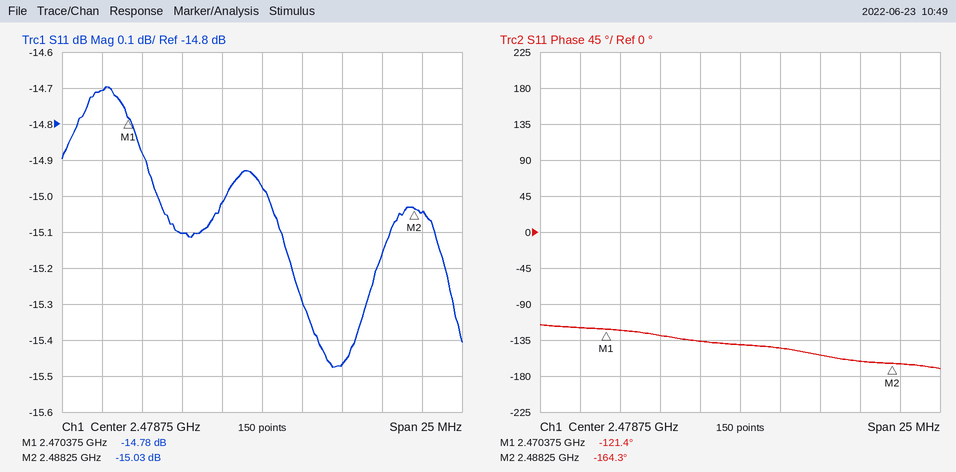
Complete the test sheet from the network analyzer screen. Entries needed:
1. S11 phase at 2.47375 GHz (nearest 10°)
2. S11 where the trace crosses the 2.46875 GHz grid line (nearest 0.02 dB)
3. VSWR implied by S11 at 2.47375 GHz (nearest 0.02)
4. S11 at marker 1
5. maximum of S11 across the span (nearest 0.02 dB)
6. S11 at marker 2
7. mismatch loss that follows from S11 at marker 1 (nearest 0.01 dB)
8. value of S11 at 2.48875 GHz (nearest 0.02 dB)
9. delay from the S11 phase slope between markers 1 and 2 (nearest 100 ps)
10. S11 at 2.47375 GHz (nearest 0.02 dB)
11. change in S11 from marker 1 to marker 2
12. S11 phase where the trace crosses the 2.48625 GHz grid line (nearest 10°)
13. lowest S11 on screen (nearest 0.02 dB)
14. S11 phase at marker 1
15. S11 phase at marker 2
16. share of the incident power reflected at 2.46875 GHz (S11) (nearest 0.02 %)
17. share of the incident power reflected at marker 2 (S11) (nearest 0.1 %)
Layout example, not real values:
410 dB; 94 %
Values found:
-130°; -14.70 dB; 1.42; -14.78 dB; -14.70 dB; -15.03 dB; 0.15 dB; -15.04 dB; 6.7 ns; -15.10 dB; -0.25 dB; -160°; -15.48 dB; -121.4°; -164.3°; 3.38 %; 3.1 %
